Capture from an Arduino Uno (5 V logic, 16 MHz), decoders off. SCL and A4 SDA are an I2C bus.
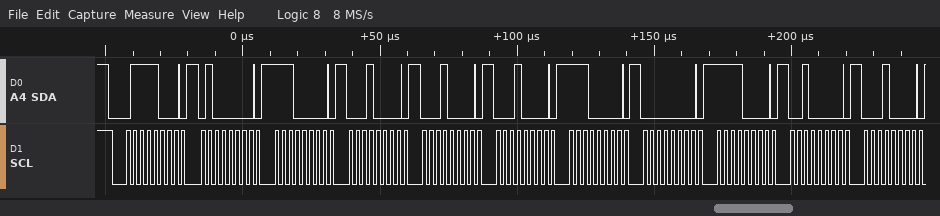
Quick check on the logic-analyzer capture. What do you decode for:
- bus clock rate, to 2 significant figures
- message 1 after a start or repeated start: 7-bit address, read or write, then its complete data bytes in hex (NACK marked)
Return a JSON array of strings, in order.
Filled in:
["400 kHz", "0x3C write: 40 E0 10 10 10 E0 00 F0 20 10"]
